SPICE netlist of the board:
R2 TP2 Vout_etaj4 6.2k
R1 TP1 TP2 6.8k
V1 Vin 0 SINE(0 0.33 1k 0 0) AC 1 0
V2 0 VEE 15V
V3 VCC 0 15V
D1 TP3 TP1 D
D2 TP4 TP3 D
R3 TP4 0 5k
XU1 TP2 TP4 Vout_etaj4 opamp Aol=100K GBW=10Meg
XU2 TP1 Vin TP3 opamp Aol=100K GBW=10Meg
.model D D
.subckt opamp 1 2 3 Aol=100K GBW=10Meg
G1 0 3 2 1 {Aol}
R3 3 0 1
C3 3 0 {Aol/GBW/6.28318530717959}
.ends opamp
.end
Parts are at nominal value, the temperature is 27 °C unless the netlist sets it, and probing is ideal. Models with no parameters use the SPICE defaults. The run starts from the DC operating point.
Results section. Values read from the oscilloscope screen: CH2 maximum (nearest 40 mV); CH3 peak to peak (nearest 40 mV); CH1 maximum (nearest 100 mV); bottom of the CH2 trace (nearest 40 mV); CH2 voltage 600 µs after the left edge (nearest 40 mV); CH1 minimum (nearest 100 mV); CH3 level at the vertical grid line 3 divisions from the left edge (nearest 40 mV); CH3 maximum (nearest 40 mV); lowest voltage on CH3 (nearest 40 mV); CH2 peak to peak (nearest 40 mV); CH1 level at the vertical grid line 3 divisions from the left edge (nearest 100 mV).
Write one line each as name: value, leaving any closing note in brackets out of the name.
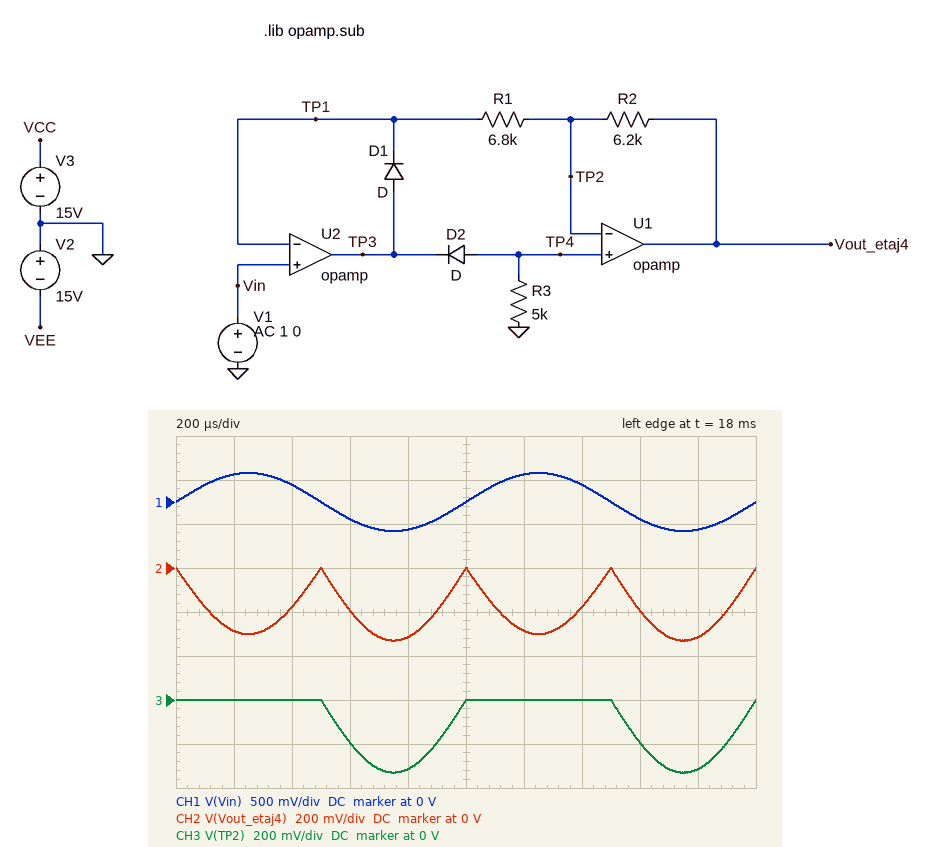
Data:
CH2 maximum: 0 V
CH3 peak to peak: 320 mV
CH1 maximum: 300 mV
bottom of the CH2 trace: -320 mV
CH2 voltage 600 µs after the left edge: -200 mV
CH1 minimum: -300 mV
CH3 level at the vertical grid line 3 divisions from the left edge: -200 mV
CH3 maximum: 0 V
lowest voltage on CH3: -320 mV
CH2 peak to peak: 320 mV
CH1 level at the vertical grid line 3 divisions from the left edge: -200 mV
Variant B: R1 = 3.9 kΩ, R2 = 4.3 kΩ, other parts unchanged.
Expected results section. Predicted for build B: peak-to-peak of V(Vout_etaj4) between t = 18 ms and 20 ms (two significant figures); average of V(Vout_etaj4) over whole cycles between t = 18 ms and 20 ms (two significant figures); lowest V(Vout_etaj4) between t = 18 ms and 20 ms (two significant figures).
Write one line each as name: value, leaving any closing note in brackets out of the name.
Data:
peak-to-peak of V(Vout_etaj4) between t = 18 ms and 20 ms: 360 mV
average of V(Vout_etaj4) over whole cycles between t = 18 ms and 20 ms: -220 mV
lowest V(Vout_etaj4) between t = 18 ms and 20 ms: -360 mV
